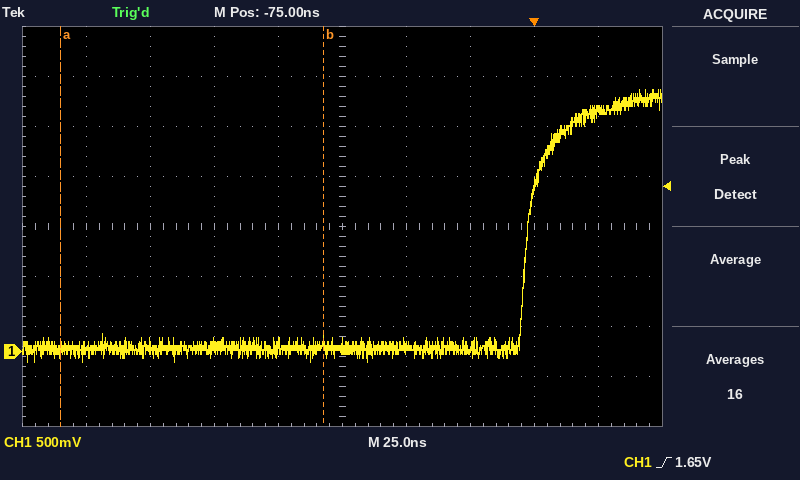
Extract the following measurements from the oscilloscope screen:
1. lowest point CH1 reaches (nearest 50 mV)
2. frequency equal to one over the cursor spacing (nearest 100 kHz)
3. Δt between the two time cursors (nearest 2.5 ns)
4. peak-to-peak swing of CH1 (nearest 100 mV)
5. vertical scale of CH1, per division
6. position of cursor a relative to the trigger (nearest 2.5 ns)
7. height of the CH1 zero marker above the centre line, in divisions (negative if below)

-100 mV
9.8 MHz
102.5 ns
2.70 V
500 mV
-185.0 ns
-2.5 div
